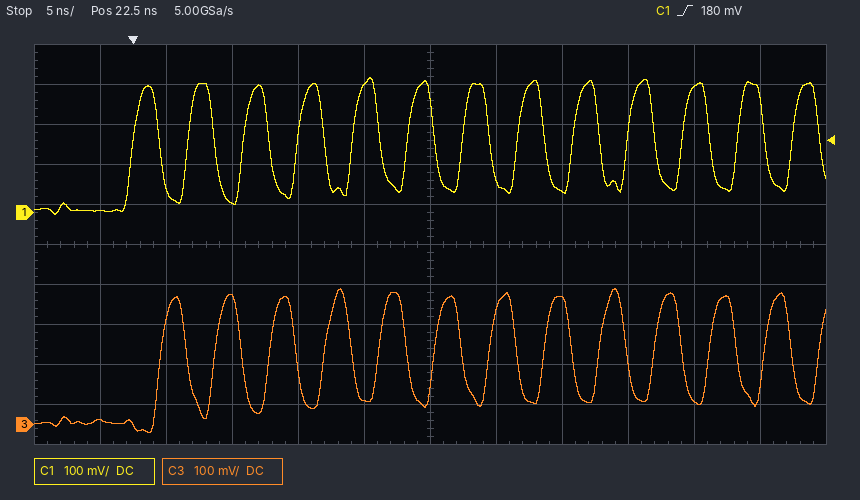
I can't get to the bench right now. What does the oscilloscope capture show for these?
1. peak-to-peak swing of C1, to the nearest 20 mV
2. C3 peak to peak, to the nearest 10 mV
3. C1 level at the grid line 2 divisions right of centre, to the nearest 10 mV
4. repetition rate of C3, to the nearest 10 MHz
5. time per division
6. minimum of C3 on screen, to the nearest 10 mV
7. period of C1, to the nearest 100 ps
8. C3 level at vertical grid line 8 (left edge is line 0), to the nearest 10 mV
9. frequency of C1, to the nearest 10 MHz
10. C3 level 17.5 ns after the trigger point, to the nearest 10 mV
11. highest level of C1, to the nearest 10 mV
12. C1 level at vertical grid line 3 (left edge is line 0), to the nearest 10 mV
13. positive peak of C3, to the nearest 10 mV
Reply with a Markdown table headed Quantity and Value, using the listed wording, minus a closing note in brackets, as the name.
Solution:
| Quantity | Value |
|---|---|
| peak-to-peak swing of C1, to the nearest 20 mV | 340 mV |
| C3 peak to peak, to the nearest 10 mV | 360 mV |
| C1 level at the grid line 2 divisions right of centre, to the nearest 10 mV | 50 mV |
| repetition rate of C3, to the nearest 10 MHz | 240 MHz |
| time per division | 5 ns |
| minimum of C3 on screen, to the nearest 10 mV | -20 mV |
| period of C1, to the nearest 100 ps | 4.2 ns |
| C3 level at vertical grid line 8 (left edge is line 0), to the nearest 10 mV | 310 mV |
| frequency of C1, to the nearest 10 MHz | 240 MHz |
| C3 level 17.5 ns after the trigger point, to the nearest 10 mV | 60 mV |
| highest level of C1, to the nearest 10 mV | 340 mV |
| C1 level at vertical grid line 3 (left edge is line 0), to the nearest 10 mV | 20 mV |
| positive peak of C3, to the nearest 10 mV | 340 mV |
